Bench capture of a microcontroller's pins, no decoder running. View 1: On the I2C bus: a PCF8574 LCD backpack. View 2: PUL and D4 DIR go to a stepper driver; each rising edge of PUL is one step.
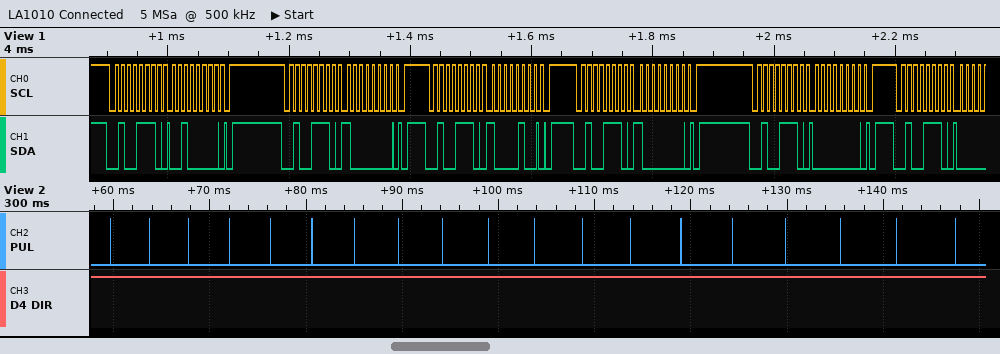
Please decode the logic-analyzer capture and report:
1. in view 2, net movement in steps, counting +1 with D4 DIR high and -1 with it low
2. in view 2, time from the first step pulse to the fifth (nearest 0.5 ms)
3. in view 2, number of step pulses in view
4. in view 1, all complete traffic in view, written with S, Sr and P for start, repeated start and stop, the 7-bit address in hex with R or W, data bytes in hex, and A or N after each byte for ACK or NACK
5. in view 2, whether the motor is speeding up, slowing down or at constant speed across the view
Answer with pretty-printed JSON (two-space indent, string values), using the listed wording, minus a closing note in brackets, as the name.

{
  "in view 2, net movement in steps, counting +1 with D4 DIR high and -1 with it low": "+19",
  "in view 2, time from the first step pulse to the fifth": "16.5 ms",
  "in view 2, number of step pulses in view": "19",
  "in view 1, all complete traffic in view, written with S, Sr and P for start, repeated start and stop, the 7-bit address in hex with R or W, data bytes in hex, and A or N after each byte for ACK or NACK": "S 27W A 20 A P S 27W A 80 A P S 27W A 84 A P S 27W A 80 A P S 27W A 00 A P S 27W A",
  "in view 2, whether the motor is speeding up, slowing down or at constant speed across the view": "slowing down"
}
